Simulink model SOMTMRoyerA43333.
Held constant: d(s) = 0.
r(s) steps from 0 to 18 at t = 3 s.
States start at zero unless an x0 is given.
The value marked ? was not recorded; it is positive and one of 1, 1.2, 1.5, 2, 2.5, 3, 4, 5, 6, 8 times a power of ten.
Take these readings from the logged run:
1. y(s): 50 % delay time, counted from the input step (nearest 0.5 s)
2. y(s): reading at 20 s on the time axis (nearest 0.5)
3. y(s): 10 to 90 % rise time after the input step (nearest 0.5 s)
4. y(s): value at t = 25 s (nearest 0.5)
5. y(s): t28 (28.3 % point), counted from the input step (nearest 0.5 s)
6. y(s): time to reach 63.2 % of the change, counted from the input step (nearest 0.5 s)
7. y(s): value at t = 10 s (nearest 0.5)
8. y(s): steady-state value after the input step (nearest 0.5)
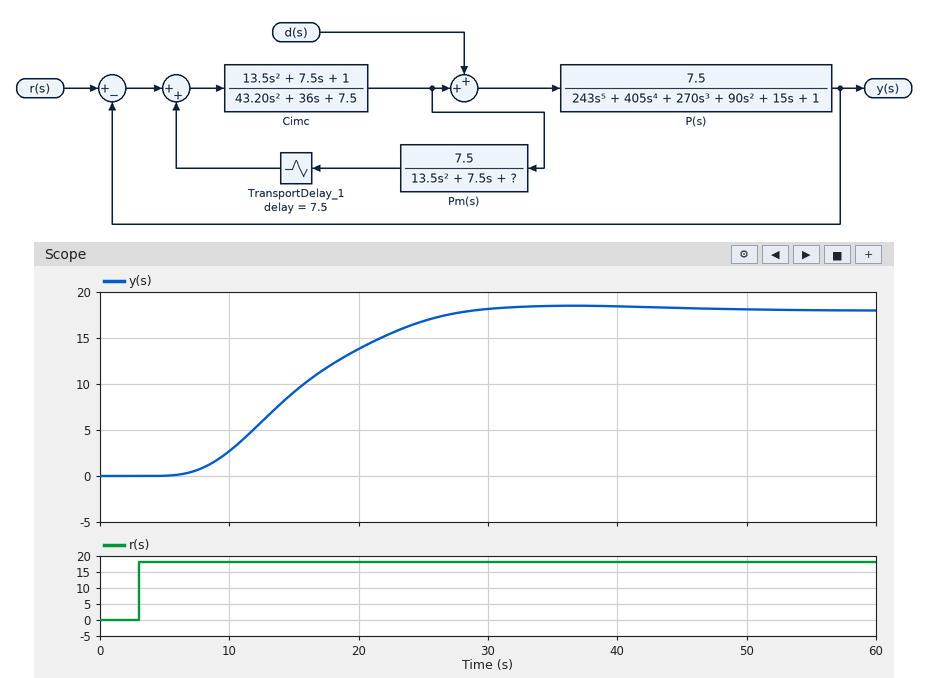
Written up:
12.0 s
14.0
14.5 s
17.0
9.0 s
14.0 s
2.5
18.0
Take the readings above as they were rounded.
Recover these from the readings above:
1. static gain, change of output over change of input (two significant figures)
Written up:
1.0
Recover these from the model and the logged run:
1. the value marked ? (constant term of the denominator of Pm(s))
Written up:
1
